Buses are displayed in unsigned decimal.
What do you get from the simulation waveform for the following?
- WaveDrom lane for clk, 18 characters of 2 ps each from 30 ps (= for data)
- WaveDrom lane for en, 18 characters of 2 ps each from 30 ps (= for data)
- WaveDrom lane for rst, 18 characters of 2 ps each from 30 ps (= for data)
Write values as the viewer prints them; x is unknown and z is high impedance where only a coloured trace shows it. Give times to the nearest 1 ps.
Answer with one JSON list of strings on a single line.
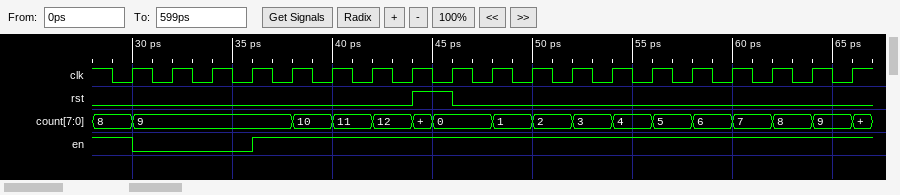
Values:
["{name: 'clk', wave: 'p.................'}", "{name: 'en', wave: '0..1..............'}", "{name: 'rst', wave: '0......10.........'}"]
